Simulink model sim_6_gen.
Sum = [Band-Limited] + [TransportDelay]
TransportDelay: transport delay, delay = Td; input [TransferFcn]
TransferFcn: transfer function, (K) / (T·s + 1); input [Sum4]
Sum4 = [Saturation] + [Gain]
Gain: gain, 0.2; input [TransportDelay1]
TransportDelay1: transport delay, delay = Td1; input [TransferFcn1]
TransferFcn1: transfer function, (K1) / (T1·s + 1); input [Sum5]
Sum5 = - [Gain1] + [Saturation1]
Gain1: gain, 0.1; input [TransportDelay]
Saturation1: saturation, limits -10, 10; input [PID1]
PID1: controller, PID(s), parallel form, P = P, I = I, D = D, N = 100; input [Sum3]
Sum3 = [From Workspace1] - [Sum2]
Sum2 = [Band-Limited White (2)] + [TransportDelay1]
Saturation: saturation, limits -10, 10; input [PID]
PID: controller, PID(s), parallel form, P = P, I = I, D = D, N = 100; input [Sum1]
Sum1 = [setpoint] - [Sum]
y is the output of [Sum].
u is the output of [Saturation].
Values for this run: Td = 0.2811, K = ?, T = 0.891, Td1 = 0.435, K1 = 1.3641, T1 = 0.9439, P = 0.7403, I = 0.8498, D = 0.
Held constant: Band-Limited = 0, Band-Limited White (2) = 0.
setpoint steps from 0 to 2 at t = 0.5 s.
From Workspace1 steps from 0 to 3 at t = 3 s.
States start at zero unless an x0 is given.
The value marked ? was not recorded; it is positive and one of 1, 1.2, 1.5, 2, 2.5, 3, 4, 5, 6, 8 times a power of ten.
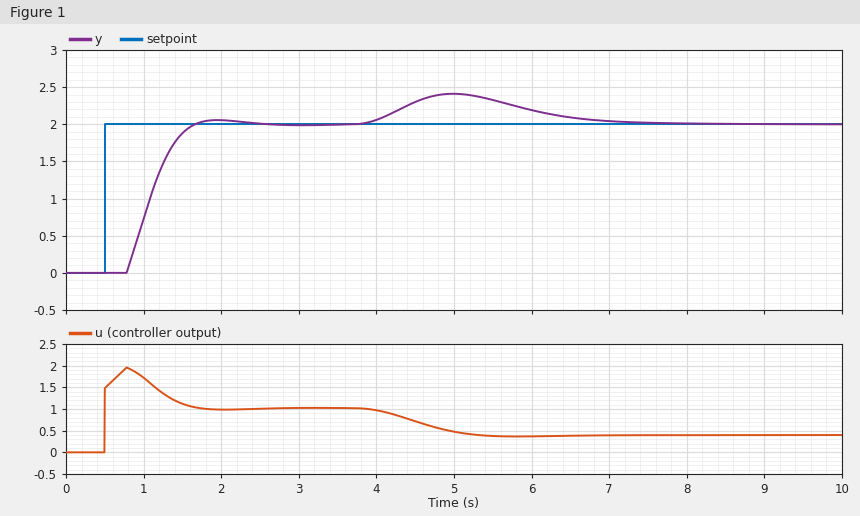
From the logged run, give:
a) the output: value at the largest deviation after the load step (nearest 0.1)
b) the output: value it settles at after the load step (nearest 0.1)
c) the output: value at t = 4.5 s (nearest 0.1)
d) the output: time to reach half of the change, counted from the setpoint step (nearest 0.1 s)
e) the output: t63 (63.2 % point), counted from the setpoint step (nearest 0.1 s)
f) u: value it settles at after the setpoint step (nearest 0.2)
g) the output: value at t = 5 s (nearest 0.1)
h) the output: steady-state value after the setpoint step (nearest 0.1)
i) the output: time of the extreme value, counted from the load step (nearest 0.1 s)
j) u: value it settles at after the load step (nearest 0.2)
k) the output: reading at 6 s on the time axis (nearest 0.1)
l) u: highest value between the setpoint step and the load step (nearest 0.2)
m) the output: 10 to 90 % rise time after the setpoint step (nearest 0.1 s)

2.4
2.0
2.3
0.6 s
0.7 s
1.0
2.4
2.0
2.0 s
0.4
2.2
2.0
0.6 s
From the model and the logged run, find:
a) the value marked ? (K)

2
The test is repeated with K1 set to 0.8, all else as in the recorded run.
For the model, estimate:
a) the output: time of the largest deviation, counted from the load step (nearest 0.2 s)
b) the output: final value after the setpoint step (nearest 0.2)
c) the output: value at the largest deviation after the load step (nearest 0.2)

2.2 s
2.0
2.2
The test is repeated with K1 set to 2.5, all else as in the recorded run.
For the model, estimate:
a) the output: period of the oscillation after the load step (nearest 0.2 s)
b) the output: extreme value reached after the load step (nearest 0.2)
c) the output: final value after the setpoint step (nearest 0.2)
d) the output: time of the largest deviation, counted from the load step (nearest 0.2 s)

2.4 s
2.6
2.0
1.8 s
